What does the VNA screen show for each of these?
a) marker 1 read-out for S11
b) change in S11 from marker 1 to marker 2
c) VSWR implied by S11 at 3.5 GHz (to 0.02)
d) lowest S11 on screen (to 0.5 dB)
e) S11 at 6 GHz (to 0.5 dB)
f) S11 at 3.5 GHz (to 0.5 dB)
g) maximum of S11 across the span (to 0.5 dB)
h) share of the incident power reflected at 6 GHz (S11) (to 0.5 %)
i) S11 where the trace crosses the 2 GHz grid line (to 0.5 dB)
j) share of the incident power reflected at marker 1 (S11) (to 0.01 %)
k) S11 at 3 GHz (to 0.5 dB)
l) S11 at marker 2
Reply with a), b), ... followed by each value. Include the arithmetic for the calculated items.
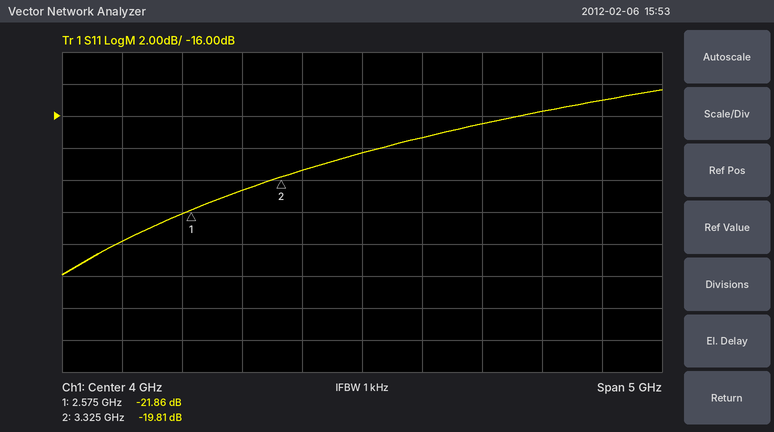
a) -21.86 dB
b) -19.81 − (-21.86) = 2.05 dB
c) |Γ| = 10^(-19.5/20) = 0.1059; VSWR = (1 + 0.1059)/(1 − 0.1059) ≈ 1.24
d) -26.0 dB
e) -15.0 dB
f) -19.5 dB
g) -14.5 dB
h) 10^(-15/10) ≈ 3.16 %, so 3.0 % to the nearest 0.5 %
i) -24.0 dB
j) 10^(-21.86/10) ≈ 0.65 %
k) -20.5 dB
l) -19.81 dB
